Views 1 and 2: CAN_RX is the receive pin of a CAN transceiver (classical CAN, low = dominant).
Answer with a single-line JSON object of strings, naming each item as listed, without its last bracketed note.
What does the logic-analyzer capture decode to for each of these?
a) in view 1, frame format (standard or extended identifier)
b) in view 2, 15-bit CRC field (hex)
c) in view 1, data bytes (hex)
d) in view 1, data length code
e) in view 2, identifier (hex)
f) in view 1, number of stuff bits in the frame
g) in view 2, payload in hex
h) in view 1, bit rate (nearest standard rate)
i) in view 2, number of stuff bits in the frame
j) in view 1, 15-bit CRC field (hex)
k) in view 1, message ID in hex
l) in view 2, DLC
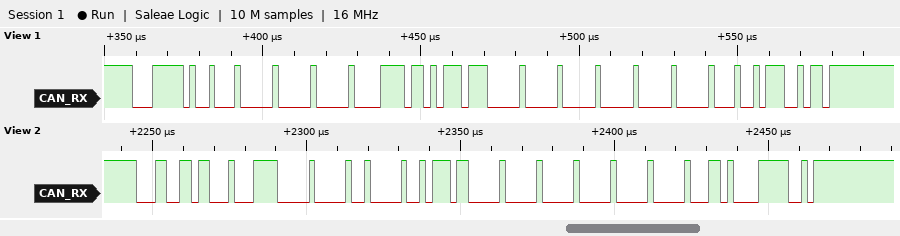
{"in view 1, frame format": "standard", "in view 2, 15-bit CRC field": "0x343E", "in view 1, data bytes": "00 00 F6 BB 80 00 00 00", "in view 1, data length code": "8", "in view 2, identifier": "0x19B", "in view 1, number of stuff bits in the frame": "10", "in view 2, payload in hex": "F0 00 80 BB 00 00 00 00", "in view 1, bit rate": "500 kbit/s", "in view 2, number of stuff bits in the frame": "10", "in view 1, 15-bit CRC field": "0x12E5", "in view 1, message ID in hex": "0x1F9", "in view 2, DLC": "8"}
